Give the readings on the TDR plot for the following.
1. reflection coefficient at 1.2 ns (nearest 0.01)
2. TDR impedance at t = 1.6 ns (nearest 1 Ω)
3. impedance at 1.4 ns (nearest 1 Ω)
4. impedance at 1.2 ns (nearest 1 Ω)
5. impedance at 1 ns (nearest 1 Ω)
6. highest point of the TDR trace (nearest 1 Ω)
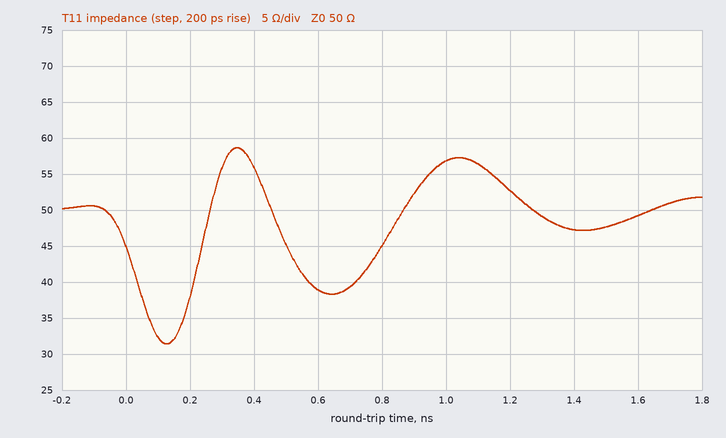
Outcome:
+0.03
49 Ω
47 Ω
53 Ω
57 Ω
59 Ω
